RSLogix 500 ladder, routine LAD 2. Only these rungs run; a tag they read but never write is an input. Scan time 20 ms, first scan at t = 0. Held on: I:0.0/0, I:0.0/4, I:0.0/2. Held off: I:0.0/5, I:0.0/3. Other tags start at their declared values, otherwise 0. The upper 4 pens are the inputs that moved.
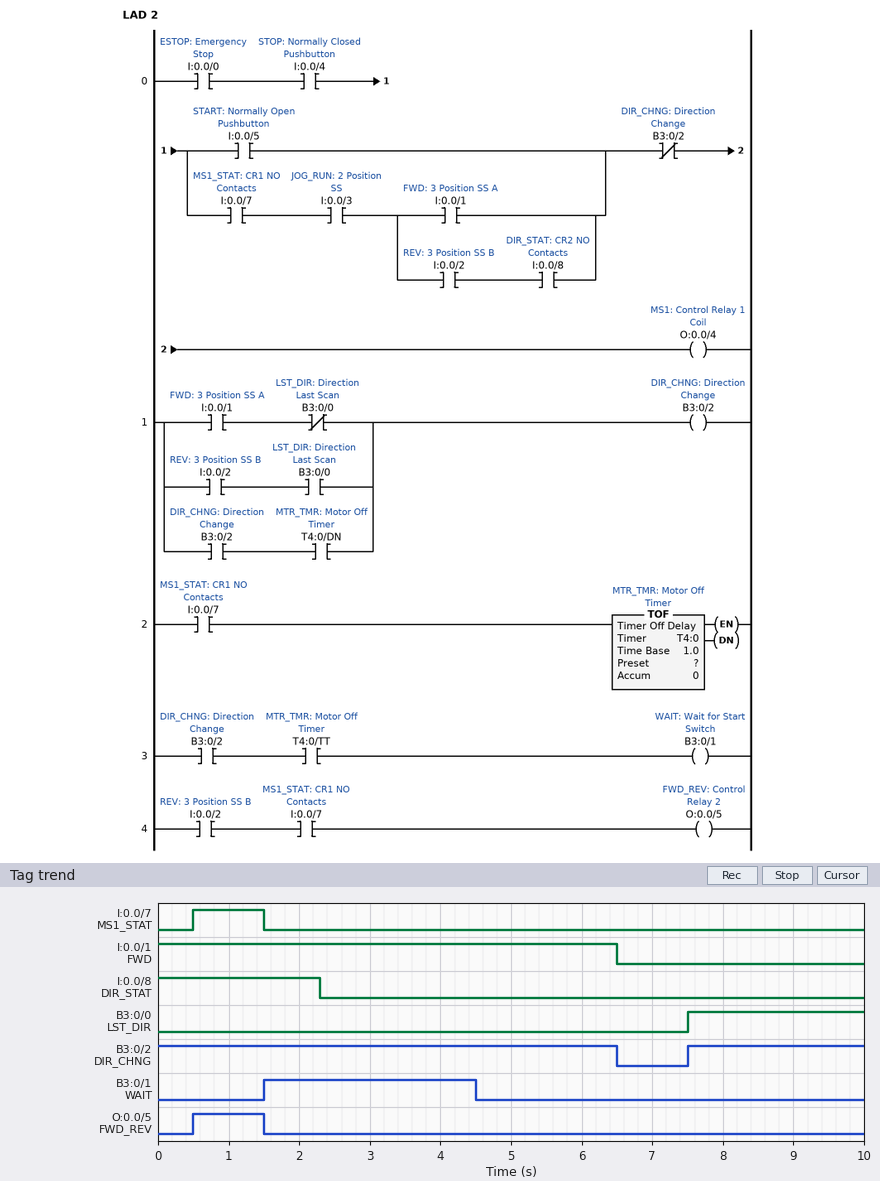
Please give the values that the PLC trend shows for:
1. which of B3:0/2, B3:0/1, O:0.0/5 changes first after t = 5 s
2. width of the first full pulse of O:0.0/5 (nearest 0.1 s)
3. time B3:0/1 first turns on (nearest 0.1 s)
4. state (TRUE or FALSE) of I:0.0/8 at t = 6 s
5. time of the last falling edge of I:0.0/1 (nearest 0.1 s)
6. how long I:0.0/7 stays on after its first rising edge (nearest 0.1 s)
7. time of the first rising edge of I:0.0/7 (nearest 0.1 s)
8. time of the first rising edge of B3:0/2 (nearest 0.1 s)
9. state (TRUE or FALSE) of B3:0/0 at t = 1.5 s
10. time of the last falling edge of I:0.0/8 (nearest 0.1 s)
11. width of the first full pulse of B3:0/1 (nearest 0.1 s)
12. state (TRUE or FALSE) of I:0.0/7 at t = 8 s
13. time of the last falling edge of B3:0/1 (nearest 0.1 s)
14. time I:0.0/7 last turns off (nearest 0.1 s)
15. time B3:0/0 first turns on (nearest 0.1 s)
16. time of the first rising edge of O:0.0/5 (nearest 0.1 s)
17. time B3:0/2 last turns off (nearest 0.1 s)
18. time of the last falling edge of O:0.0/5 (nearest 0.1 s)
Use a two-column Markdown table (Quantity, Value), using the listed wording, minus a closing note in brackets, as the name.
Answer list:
| Quantity | Value |
|---|---|
| which of B3:0/2, B3:0/1, O:0.0/5 changes first after t = 5 s | B3:0/2 |
| width of the first full pulse of O:0.0/5 | 1.0 s |
| time B3:0/1 first turns on | 1.5 s |
| state (TRUE or FALSE) of I:0.0/8 at t = 6 s | FALSE |
| time of the last falling edge of I:0.0/1 | 6.5 s |
| how long I:0.0/7 stays on after its first rising edge | 1.0 s |
| time of the first rising edge of I:0.0/7 | 0.5 s |
| time of the first rising edge of B3:0/2 | 7.5 s |
| state (TRUE or FALSE) of B3:0/0 at t = 1.5 s | FALSE |
| time of the last falling edge of I:0.0/8 | 2.3 s |
| width of the first full pulse of B3:0/1 | 3.0 s |
| state (TRUE or FALSE) of I:0.0/7 at t = 8 s | FALSE |
| time of the last falling edge of B3:0/1 | 4.5 s |
| time I:0.0/7 last turns off | 1.5 s |
| time B3:0/0 first turns on | 7.5 s |
| time of the first rising edge of O:0.0/5 | 0.5 s |
| time B3:0/2 last turns off | 6.5 s |
| time of the last falling edge of O:0.0/5 | 1.5 s |
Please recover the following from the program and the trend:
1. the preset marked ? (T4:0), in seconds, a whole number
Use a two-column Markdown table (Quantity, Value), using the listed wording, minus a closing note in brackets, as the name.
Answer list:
| Quantity | Value |
|---|---|
| the preset marked ? (T4:0), in seconds, a whole number | 3 s |
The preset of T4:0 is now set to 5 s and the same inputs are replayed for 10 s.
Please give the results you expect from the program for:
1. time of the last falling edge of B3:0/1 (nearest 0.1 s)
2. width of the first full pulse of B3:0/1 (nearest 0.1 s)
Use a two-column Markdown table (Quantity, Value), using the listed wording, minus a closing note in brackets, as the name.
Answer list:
| Quantity | Value |
|---|---|
| time of the last falling edge of B3:0/1 | 6.5 s |
| width of the first full pulse of B3:0/1 | 5.0 s |
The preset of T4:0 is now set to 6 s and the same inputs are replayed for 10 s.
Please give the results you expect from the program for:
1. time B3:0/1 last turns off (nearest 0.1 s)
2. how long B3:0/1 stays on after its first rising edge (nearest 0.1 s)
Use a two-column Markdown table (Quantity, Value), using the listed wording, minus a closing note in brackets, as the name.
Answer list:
| Quantity | Value |
|---|---|
| time B3:0/1 last turns off | 7.5 s |
| how long B3:0/1 stays on after its first rising edge | 6.0 s |
